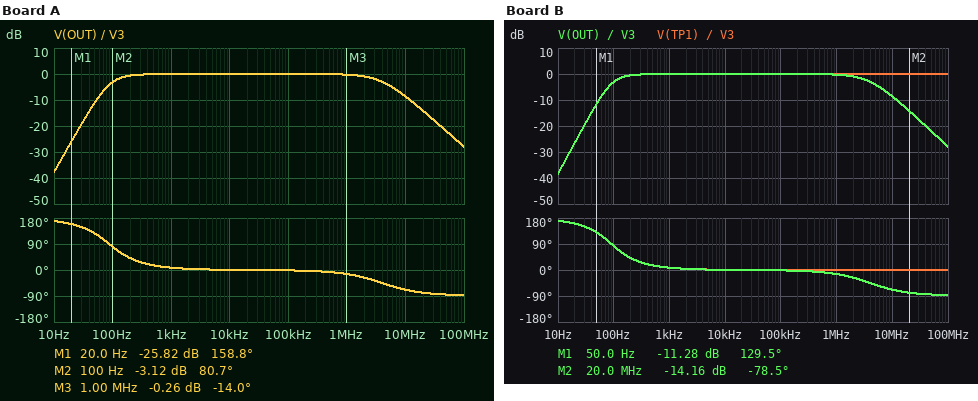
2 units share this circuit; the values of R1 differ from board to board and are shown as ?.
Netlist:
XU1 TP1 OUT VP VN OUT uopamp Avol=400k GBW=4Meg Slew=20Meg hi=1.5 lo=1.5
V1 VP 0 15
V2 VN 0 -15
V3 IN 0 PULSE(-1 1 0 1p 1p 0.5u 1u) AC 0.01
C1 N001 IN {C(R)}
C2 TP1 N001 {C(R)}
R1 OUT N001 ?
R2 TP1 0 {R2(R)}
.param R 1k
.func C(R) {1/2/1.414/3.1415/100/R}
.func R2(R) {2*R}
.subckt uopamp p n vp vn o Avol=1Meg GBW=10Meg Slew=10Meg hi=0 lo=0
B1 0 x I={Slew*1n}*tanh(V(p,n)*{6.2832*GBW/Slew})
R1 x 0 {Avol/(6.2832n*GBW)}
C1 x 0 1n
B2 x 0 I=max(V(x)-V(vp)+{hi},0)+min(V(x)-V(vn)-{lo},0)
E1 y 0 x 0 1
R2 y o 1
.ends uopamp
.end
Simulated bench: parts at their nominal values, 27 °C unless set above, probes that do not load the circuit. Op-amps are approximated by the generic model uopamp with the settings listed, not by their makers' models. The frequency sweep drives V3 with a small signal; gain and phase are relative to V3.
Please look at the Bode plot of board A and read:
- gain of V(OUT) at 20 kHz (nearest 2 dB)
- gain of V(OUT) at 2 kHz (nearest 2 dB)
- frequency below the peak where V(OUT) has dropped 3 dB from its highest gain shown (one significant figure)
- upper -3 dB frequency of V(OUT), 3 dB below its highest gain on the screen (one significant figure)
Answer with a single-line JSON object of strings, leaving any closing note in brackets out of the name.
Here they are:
{"gain of V(OUT) at 20 kHz": "0 dB", "gain of V(OUT) at 2 kHz": "0 dB", "frequency below the peak where V(OUT) has dropped 3 dB from its highest gain shown": "100 Hz", "upper -3 dB frequency of V(OUT), 3 dB below its highest gain on the screen": "4 MHz"}
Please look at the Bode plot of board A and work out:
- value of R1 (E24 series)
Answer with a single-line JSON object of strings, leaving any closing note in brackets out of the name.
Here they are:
{"value of R1": "1.3 kΩ"}
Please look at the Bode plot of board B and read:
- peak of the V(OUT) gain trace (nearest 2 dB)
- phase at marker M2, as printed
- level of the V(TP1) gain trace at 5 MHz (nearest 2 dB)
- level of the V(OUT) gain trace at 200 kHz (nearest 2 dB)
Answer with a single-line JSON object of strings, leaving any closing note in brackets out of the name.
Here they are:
{"peak of the V(OUT) gain trace": "0 dB", "phase at marker M2, as printed": "-78.5 deg", "level of the V(TP1) gain trace at 5 MHz": "0 dB", "level of the V(OUT) gain trace at 200 kHz": "0 dB"}
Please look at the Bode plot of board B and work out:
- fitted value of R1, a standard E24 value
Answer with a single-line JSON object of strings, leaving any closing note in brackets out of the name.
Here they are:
{"fitted value of R1, a standard E24 value": "1.2 kΩ"}
